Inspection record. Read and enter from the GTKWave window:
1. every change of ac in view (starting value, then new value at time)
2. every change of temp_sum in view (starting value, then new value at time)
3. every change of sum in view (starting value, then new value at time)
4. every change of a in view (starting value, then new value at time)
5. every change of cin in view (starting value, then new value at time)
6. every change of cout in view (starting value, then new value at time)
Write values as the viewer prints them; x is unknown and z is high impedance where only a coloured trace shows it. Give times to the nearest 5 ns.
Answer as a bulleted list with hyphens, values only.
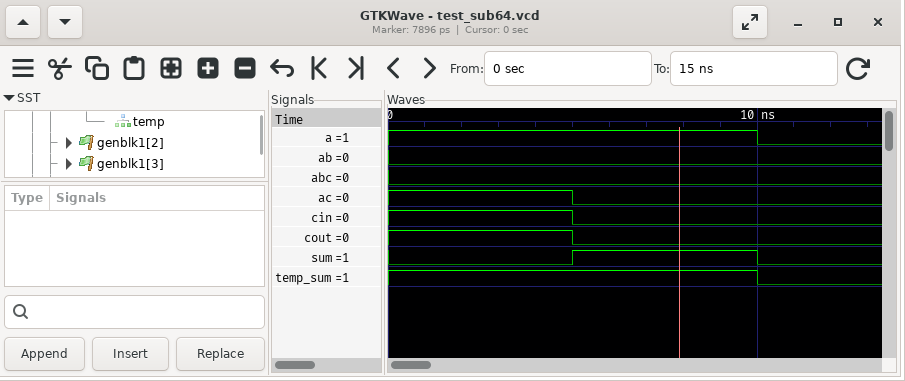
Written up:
- 1, 0 at 5 ns
- 1, 0 at 10 ns
- 0, 1 at 5 ns, 0 at 10 ns
- 1, 0 at 10 ns
- 1, 0 at 5 ns
- 1, 0 at 5 ns
